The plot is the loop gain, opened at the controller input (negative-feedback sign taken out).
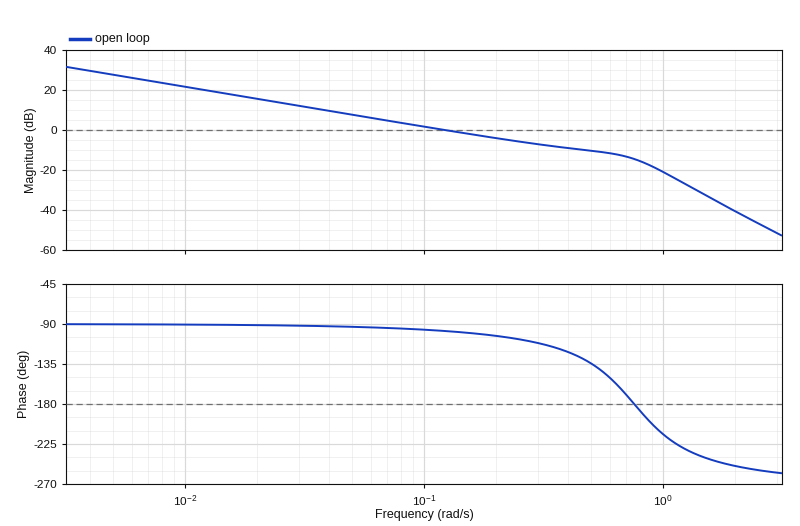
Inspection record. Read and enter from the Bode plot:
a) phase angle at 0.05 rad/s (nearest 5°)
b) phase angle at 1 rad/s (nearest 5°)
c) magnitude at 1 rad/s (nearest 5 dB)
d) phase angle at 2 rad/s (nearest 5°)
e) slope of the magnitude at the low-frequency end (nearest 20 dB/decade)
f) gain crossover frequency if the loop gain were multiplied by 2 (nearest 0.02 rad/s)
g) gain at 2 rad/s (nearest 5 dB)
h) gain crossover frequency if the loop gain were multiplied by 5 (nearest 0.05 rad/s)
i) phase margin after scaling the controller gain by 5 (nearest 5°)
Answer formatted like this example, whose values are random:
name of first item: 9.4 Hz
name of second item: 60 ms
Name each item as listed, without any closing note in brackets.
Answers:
phase angle at 0.05 rad/s: -95°
phase angle at 1 rad/s: -215°
magnitude at 1 rad/s: -20 dB
phase angle at 2 rad/s: -250°
slope of the magnitude at the low-frequency end: -20 dB/decade
gain crossover frequency if the loop gain were multiplied by 2: 0.26 rad/s
gain at 2 rad/s: -40 dB
gain crossover frequency if the loop gain were multiplied by 5: 0.75 rad/s
phase margin after scaling the controller gain by 5: 5°
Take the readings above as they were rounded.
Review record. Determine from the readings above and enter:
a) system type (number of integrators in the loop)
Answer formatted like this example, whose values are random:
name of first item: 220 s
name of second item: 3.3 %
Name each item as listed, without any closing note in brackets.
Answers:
system type: 1
